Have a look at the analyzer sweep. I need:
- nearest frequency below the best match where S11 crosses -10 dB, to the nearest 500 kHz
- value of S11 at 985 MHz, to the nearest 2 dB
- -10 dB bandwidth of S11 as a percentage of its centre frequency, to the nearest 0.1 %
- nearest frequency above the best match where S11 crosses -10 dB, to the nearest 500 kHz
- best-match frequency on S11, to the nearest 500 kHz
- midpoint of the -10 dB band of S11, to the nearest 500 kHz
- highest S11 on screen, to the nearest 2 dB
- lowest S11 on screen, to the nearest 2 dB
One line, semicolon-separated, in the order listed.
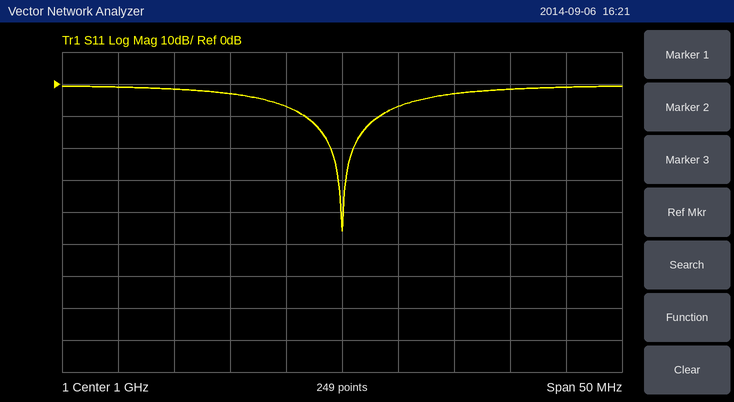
996.5 MHz; -2 dB; 0.7 %; 1.0035 GHz; 1.0000 GHz; 1.0000 GHz; 0 dB; -46 dB
